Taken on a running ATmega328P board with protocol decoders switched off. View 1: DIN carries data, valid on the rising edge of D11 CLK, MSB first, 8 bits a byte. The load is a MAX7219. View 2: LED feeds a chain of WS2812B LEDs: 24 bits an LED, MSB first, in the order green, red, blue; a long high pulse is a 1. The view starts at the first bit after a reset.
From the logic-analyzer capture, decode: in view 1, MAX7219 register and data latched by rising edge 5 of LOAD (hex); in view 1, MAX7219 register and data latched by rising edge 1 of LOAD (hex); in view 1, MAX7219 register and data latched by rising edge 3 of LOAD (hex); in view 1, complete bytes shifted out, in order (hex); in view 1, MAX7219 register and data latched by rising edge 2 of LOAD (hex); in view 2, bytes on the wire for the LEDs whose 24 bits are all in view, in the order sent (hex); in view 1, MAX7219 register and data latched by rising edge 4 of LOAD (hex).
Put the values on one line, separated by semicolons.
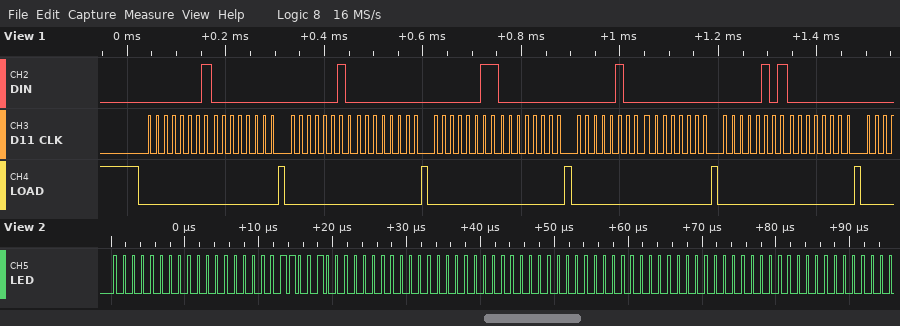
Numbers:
register 0x5, data 0x00; register 0x1, data 0x00; register 0x3, data 0x00; 0x01 0x00 0x02 0x00 0x03 0x00 0x04 0x00 0x05 0x00; register 0x2, data 0x00; 00 00 32 00 00 00 00 00 00; register 0x4, data 0x00
